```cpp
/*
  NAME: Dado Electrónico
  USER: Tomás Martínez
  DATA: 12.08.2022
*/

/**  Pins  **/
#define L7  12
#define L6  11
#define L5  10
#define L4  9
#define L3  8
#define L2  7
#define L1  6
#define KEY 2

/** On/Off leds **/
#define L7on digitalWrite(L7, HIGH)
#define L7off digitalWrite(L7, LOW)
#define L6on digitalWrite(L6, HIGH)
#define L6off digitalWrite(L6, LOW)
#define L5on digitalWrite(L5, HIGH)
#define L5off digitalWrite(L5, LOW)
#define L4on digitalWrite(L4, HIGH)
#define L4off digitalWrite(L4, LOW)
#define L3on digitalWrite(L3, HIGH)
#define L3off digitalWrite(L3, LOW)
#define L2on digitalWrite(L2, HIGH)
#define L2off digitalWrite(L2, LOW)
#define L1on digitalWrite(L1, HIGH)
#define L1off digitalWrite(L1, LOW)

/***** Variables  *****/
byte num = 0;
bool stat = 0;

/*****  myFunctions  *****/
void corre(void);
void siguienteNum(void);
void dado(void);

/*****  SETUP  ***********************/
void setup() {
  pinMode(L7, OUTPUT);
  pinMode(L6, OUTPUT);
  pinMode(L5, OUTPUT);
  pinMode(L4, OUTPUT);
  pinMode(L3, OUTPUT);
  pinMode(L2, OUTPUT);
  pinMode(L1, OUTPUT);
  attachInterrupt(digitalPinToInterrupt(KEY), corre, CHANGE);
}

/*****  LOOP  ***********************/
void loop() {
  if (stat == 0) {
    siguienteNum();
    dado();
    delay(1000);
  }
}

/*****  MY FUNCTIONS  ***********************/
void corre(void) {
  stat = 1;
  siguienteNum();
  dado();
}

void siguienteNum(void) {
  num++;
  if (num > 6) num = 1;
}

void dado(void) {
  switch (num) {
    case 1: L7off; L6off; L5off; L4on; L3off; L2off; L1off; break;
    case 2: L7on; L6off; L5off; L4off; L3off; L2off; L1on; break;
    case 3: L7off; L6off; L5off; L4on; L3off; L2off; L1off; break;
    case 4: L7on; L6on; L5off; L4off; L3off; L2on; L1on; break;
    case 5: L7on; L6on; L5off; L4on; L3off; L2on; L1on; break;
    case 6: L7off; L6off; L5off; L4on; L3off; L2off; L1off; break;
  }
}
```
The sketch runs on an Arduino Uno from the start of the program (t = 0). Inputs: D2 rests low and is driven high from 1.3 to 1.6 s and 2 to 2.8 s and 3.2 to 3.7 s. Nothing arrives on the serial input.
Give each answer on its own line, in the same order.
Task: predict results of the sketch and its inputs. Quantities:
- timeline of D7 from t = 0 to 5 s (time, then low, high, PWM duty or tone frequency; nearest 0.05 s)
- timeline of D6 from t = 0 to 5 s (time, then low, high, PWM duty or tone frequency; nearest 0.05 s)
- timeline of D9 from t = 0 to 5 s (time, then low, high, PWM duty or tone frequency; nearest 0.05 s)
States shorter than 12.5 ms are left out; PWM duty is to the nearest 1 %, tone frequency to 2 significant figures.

0 s low; 1.6 s high; 2.8 s low
0 s low; 1 s high; 1.3 s low; 1.6 s high; 2.8 s low; 3.7 s high
0 s high; 1 s low; 1.3 s high; 1.6 s low; 2 s high; 3.7 s low
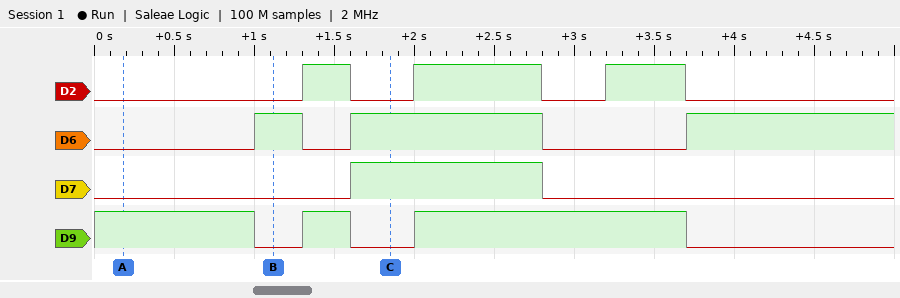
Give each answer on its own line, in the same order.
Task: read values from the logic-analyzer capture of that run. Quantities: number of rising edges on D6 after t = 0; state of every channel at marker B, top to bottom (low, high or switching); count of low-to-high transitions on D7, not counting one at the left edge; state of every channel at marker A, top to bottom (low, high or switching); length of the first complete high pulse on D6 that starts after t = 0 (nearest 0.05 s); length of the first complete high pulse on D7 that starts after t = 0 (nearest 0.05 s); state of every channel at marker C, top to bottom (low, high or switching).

3
D2 low, D6 high, D7 low, D9 low
1
D2 low, D6 low, D7 low, D9 high
0.30 s
1.20 s
D2 low, D6 high, D7 high, D9 low
